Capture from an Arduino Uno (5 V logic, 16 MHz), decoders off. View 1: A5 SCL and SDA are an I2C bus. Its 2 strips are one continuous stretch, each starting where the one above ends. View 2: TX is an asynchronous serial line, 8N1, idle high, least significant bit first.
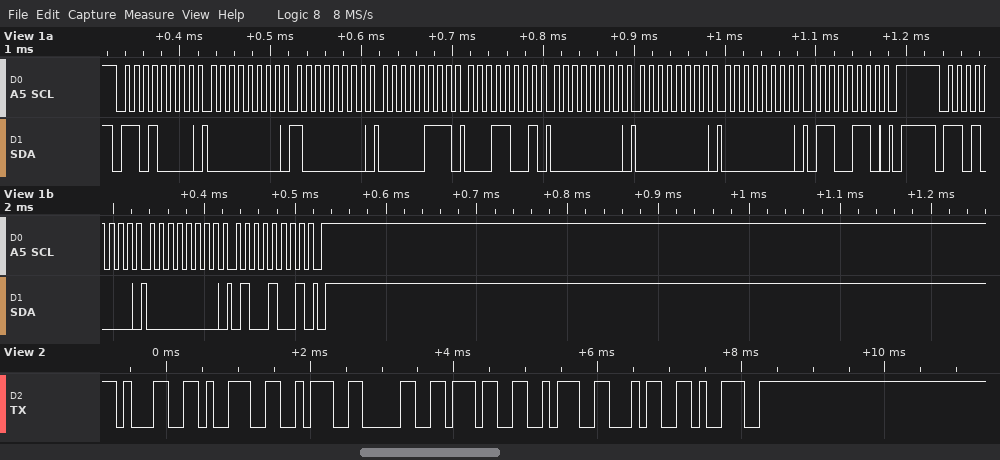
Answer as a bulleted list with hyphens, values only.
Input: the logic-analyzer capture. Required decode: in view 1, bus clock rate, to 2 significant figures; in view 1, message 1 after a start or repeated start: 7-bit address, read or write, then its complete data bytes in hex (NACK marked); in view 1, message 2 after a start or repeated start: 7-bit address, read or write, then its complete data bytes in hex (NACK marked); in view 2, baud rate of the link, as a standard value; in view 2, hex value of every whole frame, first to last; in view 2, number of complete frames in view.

- 100 kHz
- 0x68 write: 00 80 07 19 00 00 00 66
- 0x68 write: 00 49
- 9600 baud
- 0x31 0x39 0x3A 0x30 0x37 0x3A 0x34 0x39
- 8
